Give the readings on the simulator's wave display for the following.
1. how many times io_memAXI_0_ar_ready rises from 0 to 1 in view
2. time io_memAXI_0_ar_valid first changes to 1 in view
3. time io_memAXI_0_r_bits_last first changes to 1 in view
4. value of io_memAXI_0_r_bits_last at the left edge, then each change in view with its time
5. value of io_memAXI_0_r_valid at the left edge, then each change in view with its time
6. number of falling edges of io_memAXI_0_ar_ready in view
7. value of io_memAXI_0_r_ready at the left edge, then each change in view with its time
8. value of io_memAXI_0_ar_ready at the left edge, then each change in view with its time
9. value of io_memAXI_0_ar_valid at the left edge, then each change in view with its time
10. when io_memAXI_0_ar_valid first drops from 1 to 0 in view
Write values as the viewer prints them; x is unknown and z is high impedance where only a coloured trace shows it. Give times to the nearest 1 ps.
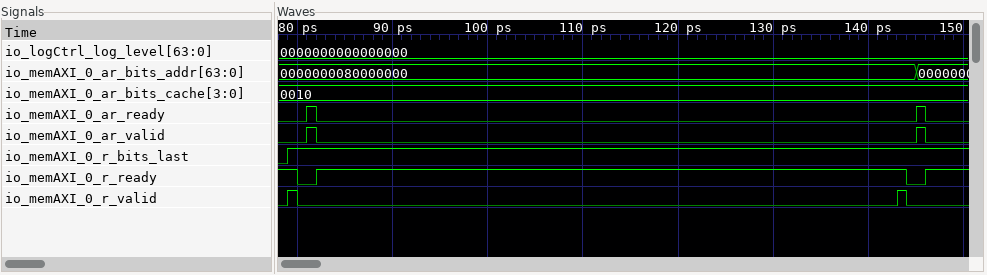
2
81 ps
79 ps
0, 1 at 79 ps
0, 1 at 79 ps, 0 at 80 ps, 1 at 143 ps, 0 at 144 ps
2
1, 0 at 80 ps, 1 at 82 ps, 0 at 144 ps, 1 at 146 ps
0, 1 at 81 ps, 0 at 82 ps, 1 at 145 ps, 0 at 146 ps
0, 1 at 81 ps, 0 at 82 ps, 1 at 145 ps, 0 at 146 ps
82 ps
